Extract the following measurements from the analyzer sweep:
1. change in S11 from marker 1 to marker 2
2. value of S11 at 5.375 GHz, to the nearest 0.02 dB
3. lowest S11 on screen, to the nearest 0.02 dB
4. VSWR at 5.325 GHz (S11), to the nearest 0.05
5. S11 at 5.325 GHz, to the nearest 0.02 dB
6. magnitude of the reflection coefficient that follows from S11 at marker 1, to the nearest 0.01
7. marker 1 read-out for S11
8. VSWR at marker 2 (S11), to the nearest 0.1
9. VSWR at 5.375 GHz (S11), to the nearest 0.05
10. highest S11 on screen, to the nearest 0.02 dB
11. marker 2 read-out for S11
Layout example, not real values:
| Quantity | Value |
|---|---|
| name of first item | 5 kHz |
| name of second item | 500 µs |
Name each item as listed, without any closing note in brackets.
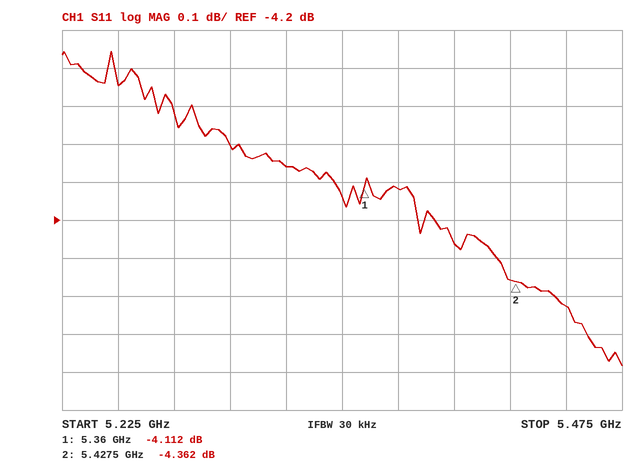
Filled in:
| Quantity | Value |
|---|---|
| change in S11 from marker 1 to marker 2 | -0.250 dB |
| value of S11 at 5.375 GHz, to the nearest 0.02 dB | -4.12 dB |
| lowest S11 on screen, to the nearest 0.02 dB | -4.58 dB |
| VSWR at 5.325 GHz (S11), to the nearest 0.05 | 4.35 |
| S11 at 5.325 GHz, to the nearest 0.02 dB | -4.06 dB |
| magnitude of the reflection coefficient that follows from S11 at marker 1, to the nearest 0.01 | 0.62 |
| marker 1 read-out for S11 | -4.112 dB |
| VSWR at marker 2 (S11), to the nearest 0.1 | 4.1 |
| VSWR at 5.375 GHz (S11), to the nearest 0.05 | 4.30 |
| highest S11 on screen, to the nearest 0.02 dB | -3.76 dB |
| marker 2 read-out for S11 | -4.362 dB |
